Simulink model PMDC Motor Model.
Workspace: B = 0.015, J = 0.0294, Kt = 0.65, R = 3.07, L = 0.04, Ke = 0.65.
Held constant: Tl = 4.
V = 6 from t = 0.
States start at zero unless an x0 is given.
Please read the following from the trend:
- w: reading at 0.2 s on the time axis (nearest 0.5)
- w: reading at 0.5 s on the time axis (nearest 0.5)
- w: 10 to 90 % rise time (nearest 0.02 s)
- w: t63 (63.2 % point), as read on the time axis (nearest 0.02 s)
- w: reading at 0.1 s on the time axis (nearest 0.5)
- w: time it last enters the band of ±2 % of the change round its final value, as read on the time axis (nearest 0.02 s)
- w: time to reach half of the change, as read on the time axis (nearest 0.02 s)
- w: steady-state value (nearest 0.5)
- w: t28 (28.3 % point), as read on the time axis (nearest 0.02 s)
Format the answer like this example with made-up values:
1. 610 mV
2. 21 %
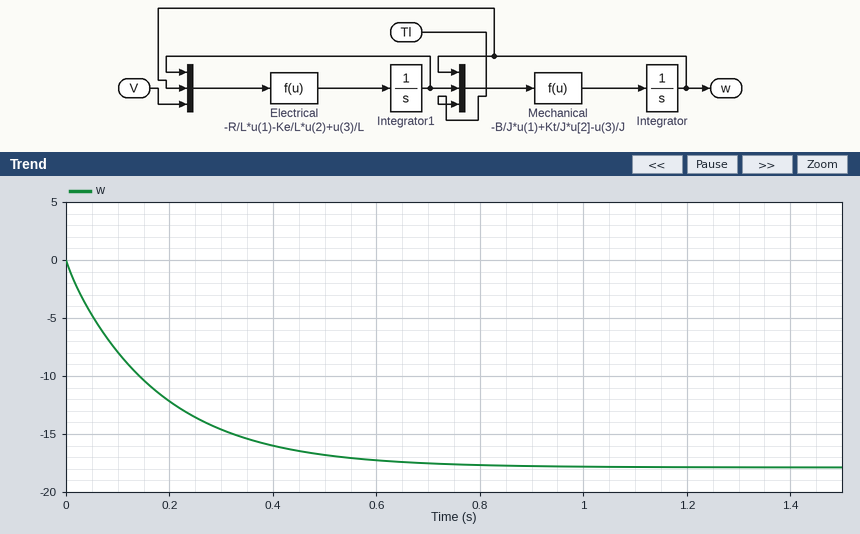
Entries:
1. -12.0
2. -17.0
3. 0.40 s
4. 0.18 s
5. -8.0
6. 0.70 s
7. 0.12 s
8. -18.0
9. 0.06 s
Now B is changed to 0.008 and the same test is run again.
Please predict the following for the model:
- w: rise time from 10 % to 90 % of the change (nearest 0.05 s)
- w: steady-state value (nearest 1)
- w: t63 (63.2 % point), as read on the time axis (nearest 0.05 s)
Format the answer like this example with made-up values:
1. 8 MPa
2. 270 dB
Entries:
1. 0.40 s
2. -19
3. 0.20 s
